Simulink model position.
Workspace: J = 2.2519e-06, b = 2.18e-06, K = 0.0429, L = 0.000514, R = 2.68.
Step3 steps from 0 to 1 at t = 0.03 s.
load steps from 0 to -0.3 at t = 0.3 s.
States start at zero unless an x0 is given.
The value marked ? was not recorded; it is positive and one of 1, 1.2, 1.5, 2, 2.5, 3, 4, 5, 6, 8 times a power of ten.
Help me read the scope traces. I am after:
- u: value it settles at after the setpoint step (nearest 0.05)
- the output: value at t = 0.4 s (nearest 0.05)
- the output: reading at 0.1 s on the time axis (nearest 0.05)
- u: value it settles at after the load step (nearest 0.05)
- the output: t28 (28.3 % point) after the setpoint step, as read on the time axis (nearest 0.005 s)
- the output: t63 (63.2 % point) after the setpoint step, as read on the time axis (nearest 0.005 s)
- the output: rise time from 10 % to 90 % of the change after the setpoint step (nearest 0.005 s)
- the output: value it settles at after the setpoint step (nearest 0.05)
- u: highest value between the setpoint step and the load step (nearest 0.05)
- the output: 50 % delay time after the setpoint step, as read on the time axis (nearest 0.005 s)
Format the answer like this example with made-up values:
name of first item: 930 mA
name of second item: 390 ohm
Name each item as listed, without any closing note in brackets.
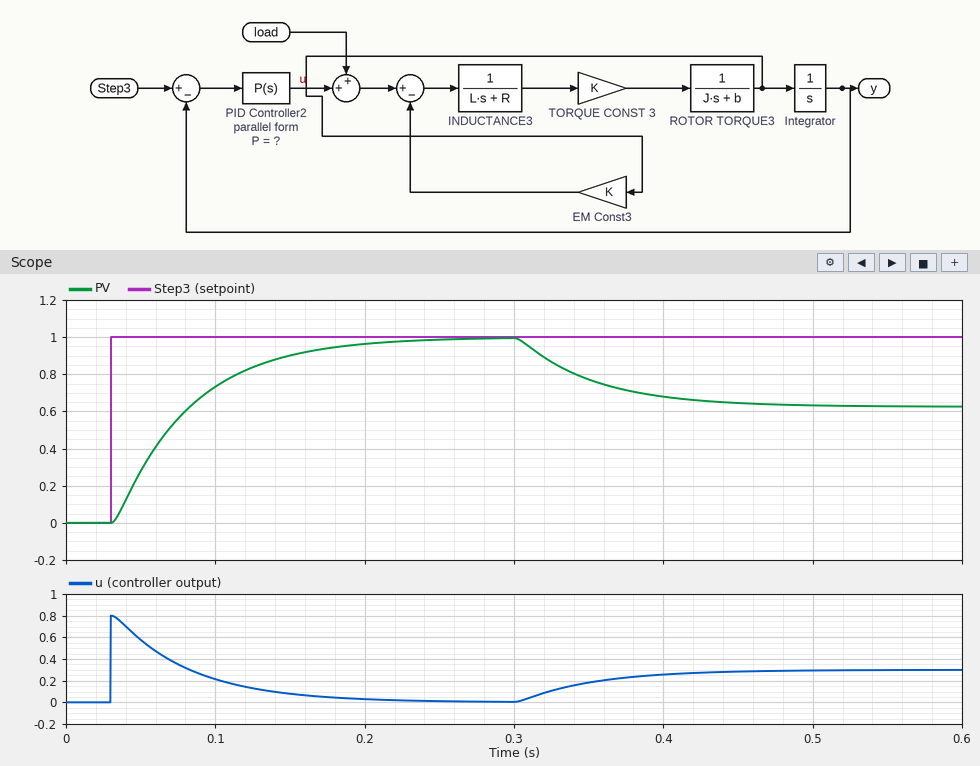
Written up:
u: value it settles at after the setpoint step: 0.00
the output: value at t = 0.4 s: 0.70
the output: reading at 0.1 s on the time axis: 0.75
u: value it settles at after the load step: 0.30
the output: t28 (28.3 % point) after the setpoint step, as read on the time axis: 0.050 s
the output: t63 (63.2 % point) after the setpoint step, as read on the time axis: 0.085 s
the output: rise time from 10 % to 90 % of the change after the setpoint step: 0.110 s
the output: value it settles at after the setpoint step: 1.00
u: highest value between the setpoint step and the load step: 0.80
the output: 50 % delay time after the setpoint step, as read on the time axis: 0.070 s
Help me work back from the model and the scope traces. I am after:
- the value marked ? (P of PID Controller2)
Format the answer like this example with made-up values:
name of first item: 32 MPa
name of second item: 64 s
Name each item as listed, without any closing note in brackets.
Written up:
the value marked ?: 0.8
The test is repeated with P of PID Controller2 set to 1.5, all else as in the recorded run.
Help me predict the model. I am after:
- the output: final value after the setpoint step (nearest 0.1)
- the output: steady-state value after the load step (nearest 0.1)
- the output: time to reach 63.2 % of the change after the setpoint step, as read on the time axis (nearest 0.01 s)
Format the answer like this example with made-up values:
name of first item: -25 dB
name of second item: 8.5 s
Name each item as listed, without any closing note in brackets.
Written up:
the output: final value after the setpoint step: 1.0
the output: steady-state value after the load step: 0.8
the output: time to reach 63.2 % of the change after the setpoint step, as read on the time axis: 0.06 s
